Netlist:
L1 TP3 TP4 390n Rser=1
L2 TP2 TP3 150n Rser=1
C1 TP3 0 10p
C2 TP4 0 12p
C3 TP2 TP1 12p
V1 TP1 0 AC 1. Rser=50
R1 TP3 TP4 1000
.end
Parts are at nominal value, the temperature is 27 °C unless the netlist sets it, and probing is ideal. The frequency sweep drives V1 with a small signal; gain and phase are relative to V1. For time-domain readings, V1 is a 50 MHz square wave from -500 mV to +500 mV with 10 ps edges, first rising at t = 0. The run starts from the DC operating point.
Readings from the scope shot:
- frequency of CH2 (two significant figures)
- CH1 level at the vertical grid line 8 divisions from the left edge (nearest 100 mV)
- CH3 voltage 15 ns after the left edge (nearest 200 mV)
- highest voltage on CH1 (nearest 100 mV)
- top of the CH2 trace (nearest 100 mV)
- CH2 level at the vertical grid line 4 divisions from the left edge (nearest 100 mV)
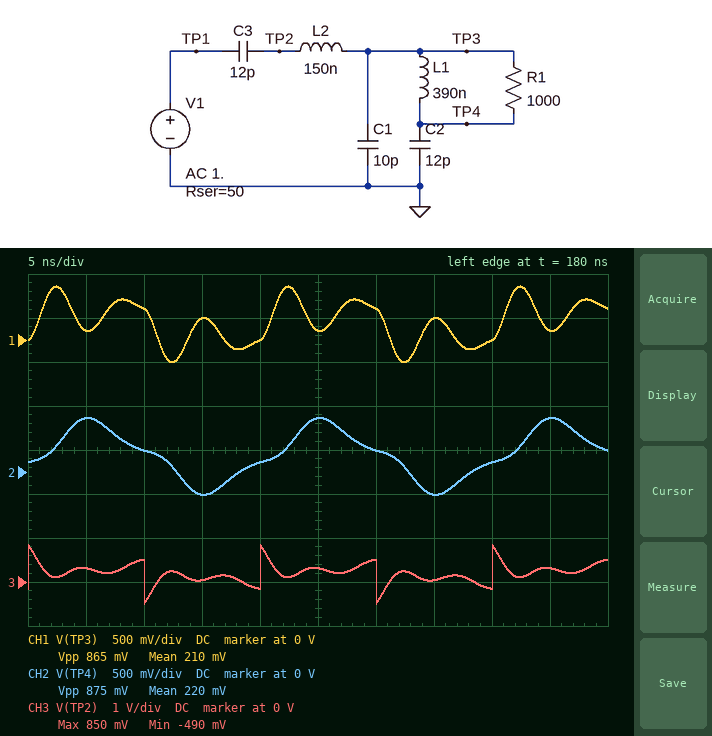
50 MHz
0 V
0 V
600 mV
600 mV
100 mV
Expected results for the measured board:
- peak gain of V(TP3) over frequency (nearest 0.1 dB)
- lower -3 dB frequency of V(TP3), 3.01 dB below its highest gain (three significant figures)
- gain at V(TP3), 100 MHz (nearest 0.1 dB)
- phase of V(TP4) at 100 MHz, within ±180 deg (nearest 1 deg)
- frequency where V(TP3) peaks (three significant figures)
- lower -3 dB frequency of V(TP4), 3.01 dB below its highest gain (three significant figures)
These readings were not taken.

4.1 dB
148 MHz
-1.6 dB
-138 deg
184 MHz
72.0 MHz
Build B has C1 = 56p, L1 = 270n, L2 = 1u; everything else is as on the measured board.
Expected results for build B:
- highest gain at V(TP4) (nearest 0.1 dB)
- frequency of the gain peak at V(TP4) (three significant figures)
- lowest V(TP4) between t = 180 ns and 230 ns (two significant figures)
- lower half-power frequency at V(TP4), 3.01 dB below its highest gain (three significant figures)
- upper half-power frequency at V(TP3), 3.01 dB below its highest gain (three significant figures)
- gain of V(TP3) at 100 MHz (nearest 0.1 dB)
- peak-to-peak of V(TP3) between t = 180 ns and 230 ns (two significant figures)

1.8 dB
49.4 MHz
-700 mV
45.4 MHz
53.0 MHz
-21.0 dB
1.1 V
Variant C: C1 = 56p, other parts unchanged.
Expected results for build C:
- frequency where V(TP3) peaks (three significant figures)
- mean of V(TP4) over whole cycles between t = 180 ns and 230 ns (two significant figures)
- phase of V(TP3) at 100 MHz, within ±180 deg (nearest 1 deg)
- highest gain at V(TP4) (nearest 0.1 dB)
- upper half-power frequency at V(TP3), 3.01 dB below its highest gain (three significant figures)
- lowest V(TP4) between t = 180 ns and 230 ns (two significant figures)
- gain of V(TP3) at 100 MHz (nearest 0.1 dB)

125 MHz
75 mV
-28 deg
0.4 dB
150 MHz
-120 mV
-8.3 dB
